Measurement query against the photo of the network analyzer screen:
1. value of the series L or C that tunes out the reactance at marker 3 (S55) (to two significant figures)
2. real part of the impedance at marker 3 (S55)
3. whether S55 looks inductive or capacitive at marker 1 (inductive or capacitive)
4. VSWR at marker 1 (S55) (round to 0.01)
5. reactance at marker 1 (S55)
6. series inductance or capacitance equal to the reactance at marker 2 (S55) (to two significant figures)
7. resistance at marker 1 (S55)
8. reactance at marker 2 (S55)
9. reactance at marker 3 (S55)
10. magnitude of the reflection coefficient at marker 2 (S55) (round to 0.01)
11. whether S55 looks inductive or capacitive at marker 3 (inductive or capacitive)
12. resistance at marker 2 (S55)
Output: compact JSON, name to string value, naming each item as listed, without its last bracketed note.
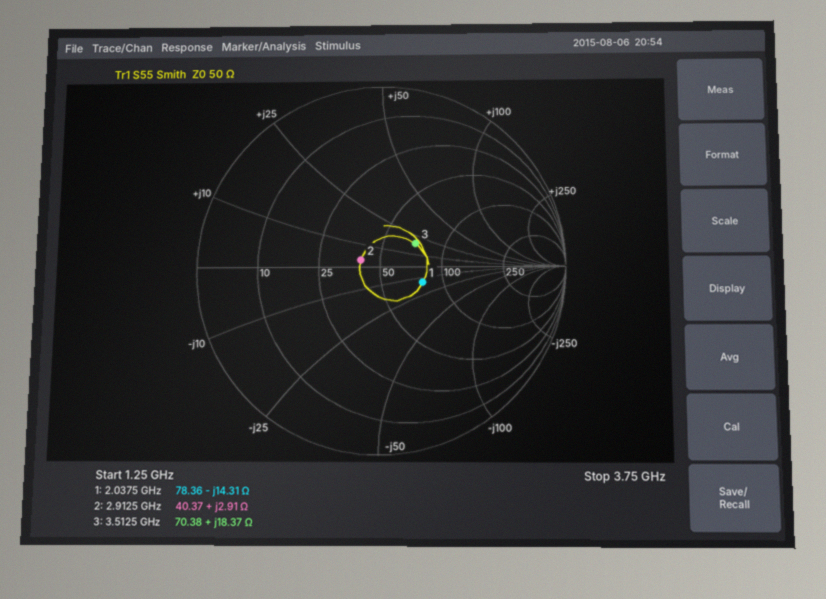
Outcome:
{"value of the series L or C that tunes out the reactance at marker 3 (S55)": "2.5 pF", "real part of the impedance at marker 3": "70.38 Ω", "whether S55 looks inductive or capacitive at marker 1": "capacitive", "VSWR at marker 1 (S55)": "1.65", "reactance at marker 1": "-14.31 Ω", "series inductance or capacitance equal to the reactance at marker 2 (S55)": "160 pH", "resistance at marker 1": "78.36 Ω", "reactance at marker 2": "+2.91 Ω", "reactance at marker 3": "+18.37 Ω", "magnitude of the reflection coefficient at marker 2 (S55)": "0.11", "whether S55 looks inductive or capacitive at marker 3": "inductive", "resistance at marker 2": "40.37 Ω"}
